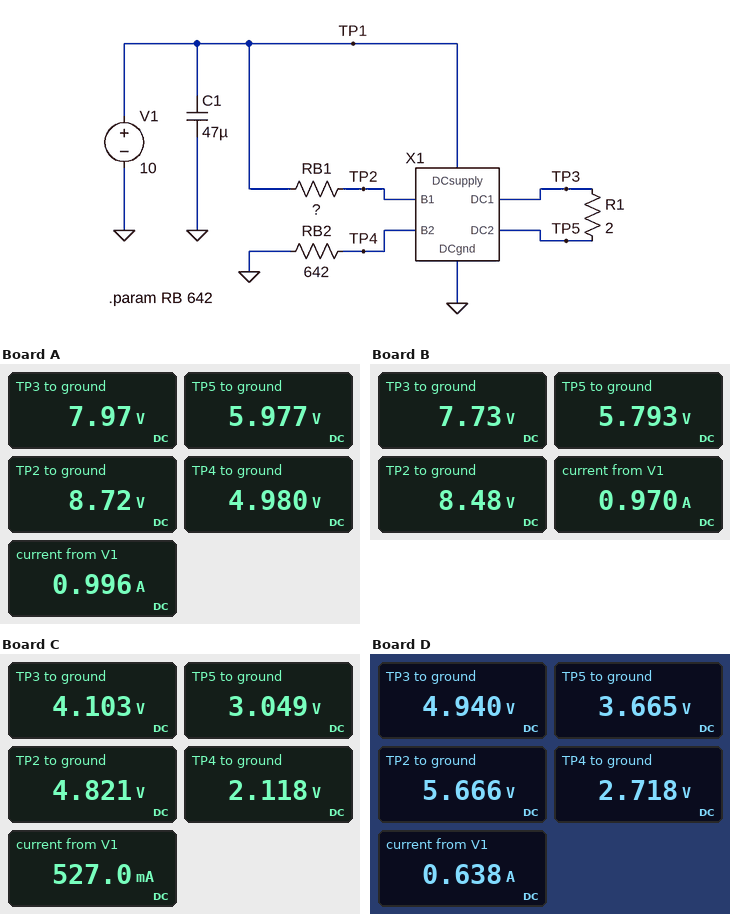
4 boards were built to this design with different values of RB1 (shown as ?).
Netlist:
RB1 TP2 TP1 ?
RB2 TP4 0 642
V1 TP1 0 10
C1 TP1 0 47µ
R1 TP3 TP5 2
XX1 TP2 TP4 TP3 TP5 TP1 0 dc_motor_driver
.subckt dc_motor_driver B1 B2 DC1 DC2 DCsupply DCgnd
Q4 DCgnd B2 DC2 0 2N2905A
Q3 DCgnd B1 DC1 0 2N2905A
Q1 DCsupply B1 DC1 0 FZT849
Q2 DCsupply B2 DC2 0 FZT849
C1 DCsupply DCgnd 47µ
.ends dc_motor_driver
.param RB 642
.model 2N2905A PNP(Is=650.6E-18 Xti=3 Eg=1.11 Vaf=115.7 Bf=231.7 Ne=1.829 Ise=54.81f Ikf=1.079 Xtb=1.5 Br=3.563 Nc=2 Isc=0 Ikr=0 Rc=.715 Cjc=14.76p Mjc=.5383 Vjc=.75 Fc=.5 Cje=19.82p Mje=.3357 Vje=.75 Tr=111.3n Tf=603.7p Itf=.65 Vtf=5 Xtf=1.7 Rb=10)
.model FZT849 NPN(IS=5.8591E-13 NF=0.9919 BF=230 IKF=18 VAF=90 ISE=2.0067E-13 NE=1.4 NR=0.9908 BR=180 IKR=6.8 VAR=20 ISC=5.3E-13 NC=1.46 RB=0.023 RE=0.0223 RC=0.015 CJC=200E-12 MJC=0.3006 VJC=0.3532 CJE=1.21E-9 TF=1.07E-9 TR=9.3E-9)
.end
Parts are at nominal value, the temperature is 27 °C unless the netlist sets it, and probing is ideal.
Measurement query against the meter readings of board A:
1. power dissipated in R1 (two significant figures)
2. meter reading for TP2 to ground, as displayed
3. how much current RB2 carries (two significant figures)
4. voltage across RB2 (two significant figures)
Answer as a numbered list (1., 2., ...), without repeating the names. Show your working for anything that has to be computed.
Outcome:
1. (7.97 V - 5.977 V)^2 / 2 Ω = 2.0 W
2. 8.72 V
3. (4.98 V) / 642 Ω = 7.8 mA
4. 4.98 V = 5.0 V
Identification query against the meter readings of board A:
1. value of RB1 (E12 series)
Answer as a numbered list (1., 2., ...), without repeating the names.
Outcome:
1. 270 Ω
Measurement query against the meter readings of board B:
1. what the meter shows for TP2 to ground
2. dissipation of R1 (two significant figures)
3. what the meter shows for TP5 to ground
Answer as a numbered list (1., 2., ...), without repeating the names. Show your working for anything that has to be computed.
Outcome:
1. 8.48 V
2. (7.73 V - 5.793 V)^2 / 2 Ω = 1.9 W
3. 5.793 V
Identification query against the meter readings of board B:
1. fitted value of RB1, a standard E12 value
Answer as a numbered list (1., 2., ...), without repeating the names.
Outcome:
1. 330 Ω
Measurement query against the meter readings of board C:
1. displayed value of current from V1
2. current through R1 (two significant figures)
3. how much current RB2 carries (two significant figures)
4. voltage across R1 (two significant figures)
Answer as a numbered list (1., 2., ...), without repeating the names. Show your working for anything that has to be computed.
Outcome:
1. 527.0 mA
2. (4.103 V - 3.049 V) / 2 Ω = 530 mA
3. (2.118 V) / 642 Ω = 3.3 mA
4. 4.103 V - 3.049 V = 1.1 V
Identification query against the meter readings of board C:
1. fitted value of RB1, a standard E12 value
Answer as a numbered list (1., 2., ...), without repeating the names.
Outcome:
1. 2.2 kΩ
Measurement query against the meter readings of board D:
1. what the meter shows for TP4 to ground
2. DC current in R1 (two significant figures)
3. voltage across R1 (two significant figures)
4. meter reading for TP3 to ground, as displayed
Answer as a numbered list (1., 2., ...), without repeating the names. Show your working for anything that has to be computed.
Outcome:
1. 2.718 V
2. (4.94 V - 3.665 V) / 2 Ω = 640 mA
3. 4.94 V - 3.665 V = 1.3 V
4. 4.940 V
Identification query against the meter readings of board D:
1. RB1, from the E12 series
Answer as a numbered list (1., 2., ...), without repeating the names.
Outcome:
1. 1.5 kΩ
